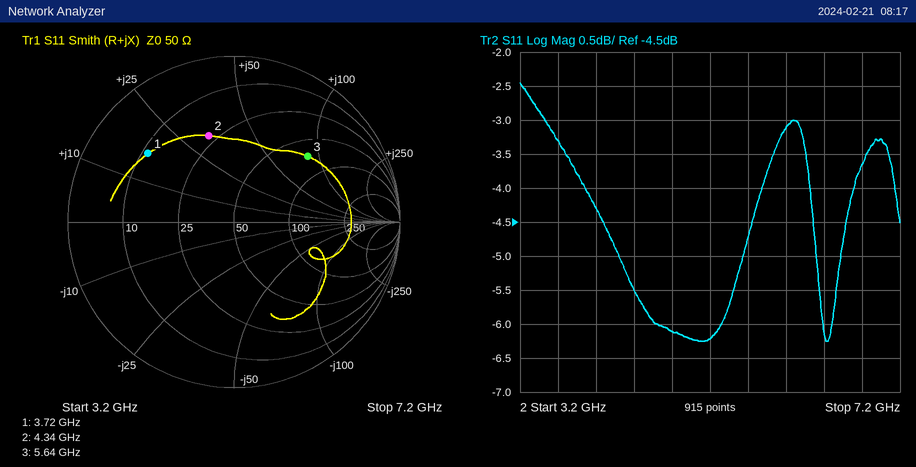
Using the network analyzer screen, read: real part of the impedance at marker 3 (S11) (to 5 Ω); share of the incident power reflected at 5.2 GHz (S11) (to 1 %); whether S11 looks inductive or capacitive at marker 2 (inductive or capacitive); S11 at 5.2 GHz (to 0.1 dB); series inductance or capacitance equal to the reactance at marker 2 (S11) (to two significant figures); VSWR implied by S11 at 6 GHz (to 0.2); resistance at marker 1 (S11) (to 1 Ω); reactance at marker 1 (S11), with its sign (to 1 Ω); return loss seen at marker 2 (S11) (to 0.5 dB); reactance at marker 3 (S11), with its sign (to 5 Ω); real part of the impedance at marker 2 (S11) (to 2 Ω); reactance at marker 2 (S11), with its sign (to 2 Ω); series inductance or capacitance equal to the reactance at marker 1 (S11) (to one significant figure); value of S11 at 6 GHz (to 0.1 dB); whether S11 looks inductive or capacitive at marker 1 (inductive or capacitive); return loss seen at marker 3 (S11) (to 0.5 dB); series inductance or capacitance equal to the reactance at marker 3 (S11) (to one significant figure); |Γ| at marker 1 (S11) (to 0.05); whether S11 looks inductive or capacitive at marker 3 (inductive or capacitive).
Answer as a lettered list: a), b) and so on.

a) 70 Ω
b) 24 %
c) inductive
d) -6.2 dB
e) 1.2 nH
f) 5.6
g) 11 Ω
h) +17 Ω
i) 5.5 dB
j) +85 Ω
k) 22 Ω
l) +32 Ω
m) 700 pH
n) -3.1 dB
o) inductive
p) 4.5 dB
q) 2 nH
r) 0.65
s) inductive
